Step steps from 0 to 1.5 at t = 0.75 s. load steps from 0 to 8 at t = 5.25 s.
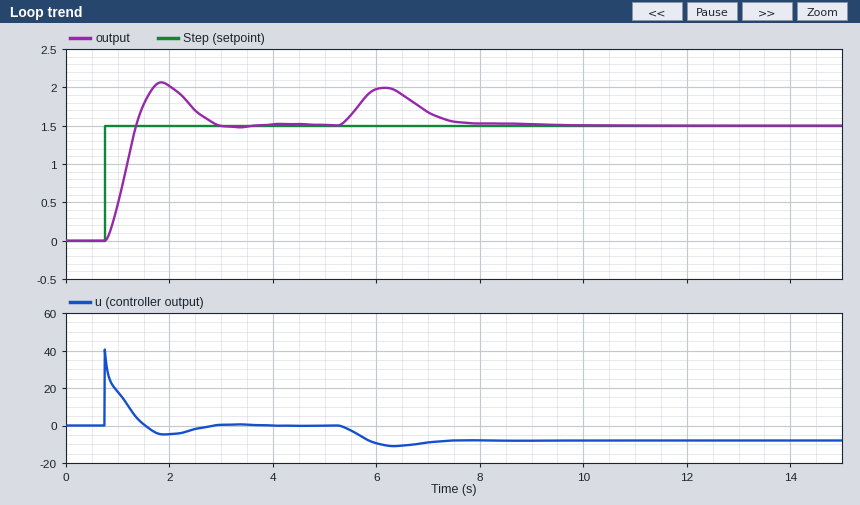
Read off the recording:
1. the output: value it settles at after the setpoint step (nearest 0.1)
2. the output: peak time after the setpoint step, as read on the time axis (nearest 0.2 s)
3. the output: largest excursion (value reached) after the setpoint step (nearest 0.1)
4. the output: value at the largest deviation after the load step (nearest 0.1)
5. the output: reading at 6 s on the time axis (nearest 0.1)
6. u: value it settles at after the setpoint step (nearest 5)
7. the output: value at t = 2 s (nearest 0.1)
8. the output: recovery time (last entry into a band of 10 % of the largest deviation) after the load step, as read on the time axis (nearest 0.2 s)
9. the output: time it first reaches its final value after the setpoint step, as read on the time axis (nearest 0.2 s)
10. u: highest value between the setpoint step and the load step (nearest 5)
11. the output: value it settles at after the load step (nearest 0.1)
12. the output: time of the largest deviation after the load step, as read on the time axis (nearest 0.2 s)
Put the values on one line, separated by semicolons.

1.5; 1.8 s; 2.1; 2.0; 2.0; 0; 2.0; 7.6 s; 1.4 s; 40; 1.5; 6.2 s
